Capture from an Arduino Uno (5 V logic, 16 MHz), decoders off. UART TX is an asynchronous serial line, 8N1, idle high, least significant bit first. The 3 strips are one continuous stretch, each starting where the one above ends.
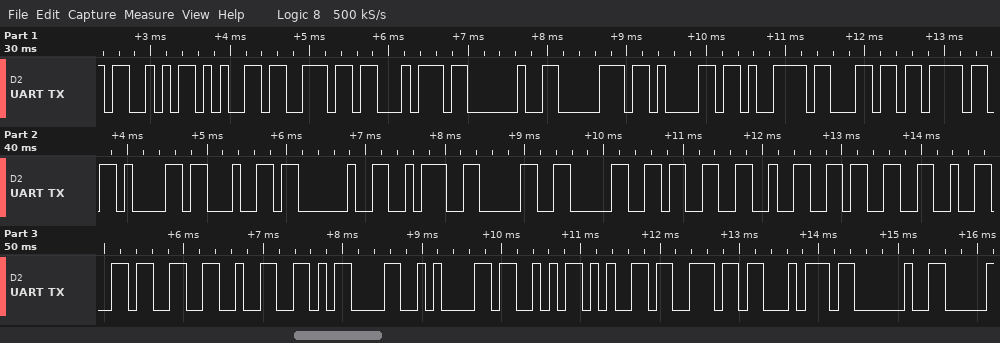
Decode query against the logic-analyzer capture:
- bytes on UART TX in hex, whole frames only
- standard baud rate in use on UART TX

53 65 6E 74 20 70 61 79 6C 6F 61 64 20 3A 30 30 33 32 33 32 33 32 0D 0A 53 65 6E 74 20
9600 baud
